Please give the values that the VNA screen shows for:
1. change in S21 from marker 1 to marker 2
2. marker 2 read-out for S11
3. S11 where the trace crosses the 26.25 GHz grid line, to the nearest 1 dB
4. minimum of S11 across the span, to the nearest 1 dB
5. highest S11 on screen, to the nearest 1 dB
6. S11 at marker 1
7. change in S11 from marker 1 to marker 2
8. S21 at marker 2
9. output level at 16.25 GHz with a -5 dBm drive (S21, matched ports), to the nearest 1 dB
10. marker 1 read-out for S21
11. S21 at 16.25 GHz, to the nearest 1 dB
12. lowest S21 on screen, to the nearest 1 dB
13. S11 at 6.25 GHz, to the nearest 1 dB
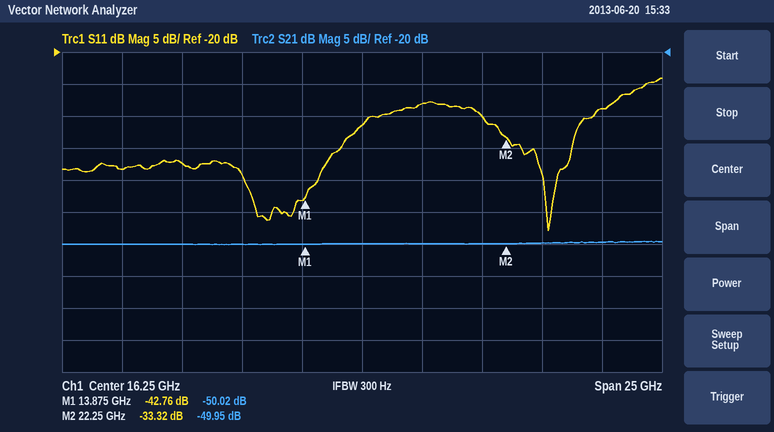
0.07 dB
-33.32 dB
-29 dB
-48 dB
-24 dB
-42.76 dB
9.44 dB
-49.95 dB
-55 dBm
-50.02 dB
-50 dB
-50 dB
-38 dB
